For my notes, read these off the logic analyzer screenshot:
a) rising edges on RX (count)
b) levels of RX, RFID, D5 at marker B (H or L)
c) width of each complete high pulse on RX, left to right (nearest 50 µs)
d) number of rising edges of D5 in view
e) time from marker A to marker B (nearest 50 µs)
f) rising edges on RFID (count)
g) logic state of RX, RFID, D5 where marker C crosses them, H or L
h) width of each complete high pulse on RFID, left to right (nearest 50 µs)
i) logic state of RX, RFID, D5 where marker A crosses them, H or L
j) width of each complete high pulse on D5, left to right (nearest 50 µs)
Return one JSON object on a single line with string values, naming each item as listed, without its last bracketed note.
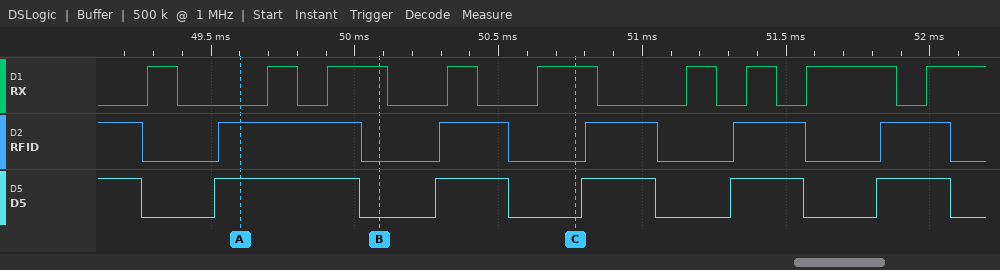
{"rising edges on RX": "9", "levels of RX, RFID, D5 at marker B": "RX=H, RFID=L, D5=L", "width of each complete high pulse on RX, left to right": "100 µs, 100 µs, 200 µs, 100 µs, 200 µs, 100 µs, 100 µs, 300 µs", "number of rising edges of D5 in view": "5", "time from marker A to marker B": "500 µs", "rising edges on RFID": "5", "logic state of RX, RFID, D5 where marker C crosses them, H or L": "RX=H, RFID=L, D5=L", "width of each complete high pulse on RFID, left to right": "500 µs, 250 µs, 250 µs, 250 µs, 250 µs", "logic state of RX, RFID, D5 where marker A crosses them, H or L": "RX=L, RFID=H, D5=H", "width of each complete high pulse on D5, left to right": "500 µs, 250 µs, 250 µs, 250 µs, 250 µs"}
